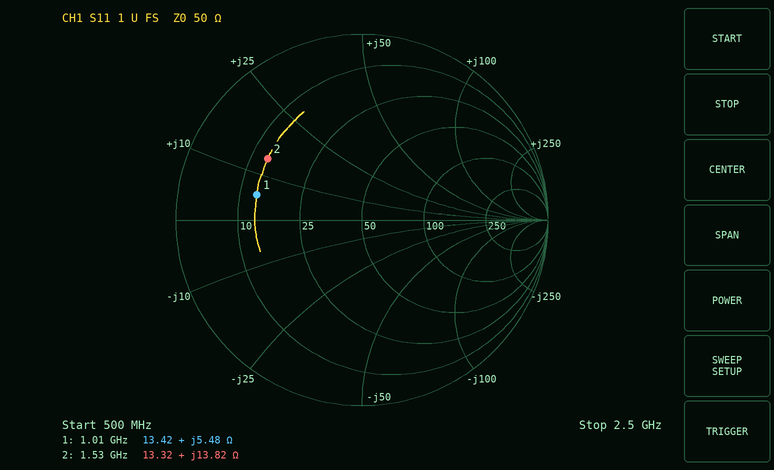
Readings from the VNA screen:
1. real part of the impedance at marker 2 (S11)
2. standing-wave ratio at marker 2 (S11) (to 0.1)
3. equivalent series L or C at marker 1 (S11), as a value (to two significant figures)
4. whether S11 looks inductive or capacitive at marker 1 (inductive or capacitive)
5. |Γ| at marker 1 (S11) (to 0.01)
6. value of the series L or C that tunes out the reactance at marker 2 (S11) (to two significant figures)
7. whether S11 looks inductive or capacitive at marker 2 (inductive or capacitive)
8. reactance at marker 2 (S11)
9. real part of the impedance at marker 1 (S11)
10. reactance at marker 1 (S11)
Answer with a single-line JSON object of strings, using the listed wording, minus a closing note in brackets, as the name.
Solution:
{"real part of the impedance at marker 2": "13.32 Ω", "standing-wave ratio at marker 2 (S11)": "4.1", "equivalent series L or C at marker 1 (S11), as a value": "860 pH", "whether S11 looks inductive or capacitive at marker 1": "inductive", "|Γ| at marker 1 (S11)": "0.58", "value of the series L or C that tunes out the reactance at marker 2 (S11)": "7.5 pF", "whether S11 looks inductive or capacitive at marker 2": "inductive", "reactance at marker 2": "+13.82 Ω", "real part of the impedance at marker 1": "13.42 Ω", "reactance at marker 1": "+5.48 Ω"}
